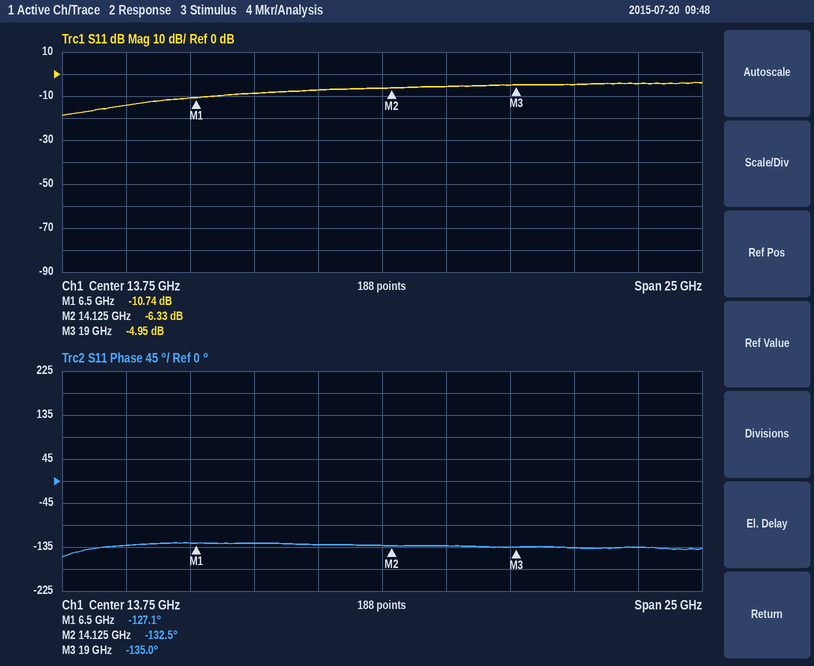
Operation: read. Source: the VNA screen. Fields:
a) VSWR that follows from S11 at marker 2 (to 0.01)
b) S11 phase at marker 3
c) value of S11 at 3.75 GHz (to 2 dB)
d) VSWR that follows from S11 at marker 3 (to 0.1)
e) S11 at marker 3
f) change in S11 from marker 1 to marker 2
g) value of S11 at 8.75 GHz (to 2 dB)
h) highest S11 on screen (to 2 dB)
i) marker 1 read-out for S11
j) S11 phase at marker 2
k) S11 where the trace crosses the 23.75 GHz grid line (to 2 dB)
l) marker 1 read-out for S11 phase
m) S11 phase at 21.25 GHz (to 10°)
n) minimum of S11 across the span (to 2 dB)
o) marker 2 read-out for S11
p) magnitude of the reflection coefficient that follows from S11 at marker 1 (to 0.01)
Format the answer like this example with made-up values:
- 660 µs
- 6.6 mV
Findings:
- 2.86
- -135.0°
- -14 dB
- 3.6
- -4.95 dB
- 4.41 dB
- -8 dB
- -4 dB
- -10.74 dB
- -132.5°
- -4 dB
- -127.1°
- -140°
- -18 dB
- -6.33 dB
- 0.29
